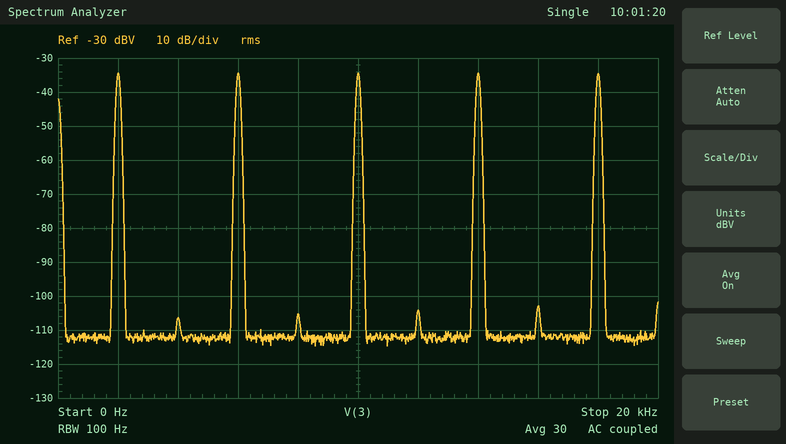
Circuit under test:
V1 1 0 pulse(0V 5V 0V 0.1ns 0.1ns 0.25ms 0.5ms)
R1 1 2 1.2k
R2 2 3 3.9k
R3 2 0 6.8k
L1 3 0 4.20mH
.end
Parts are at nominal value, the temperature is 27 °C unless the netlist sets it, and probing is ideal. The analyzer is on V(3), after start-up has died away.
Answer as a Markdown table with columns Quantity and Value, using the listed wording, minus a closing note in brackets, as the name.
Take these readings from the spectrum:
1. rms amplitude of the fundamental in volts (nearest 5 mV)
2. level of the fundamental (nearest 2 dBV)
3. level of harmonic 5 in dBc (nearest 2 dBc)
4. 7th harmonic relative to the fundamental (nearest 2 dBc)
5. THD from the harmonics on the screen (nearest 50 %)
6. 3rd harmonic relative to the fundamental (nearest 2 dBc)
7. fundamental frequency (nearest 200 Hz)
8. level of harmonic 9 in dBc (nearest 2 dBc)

| Quantity | Value |
|---|---|
| rms amplitude of the fundamental in volts | 20 mV |
| level of the fundamental | -34 dBV |
| level of harmonic 5 in dBc | 0 dBc |
| 7th harmonic relative to the fundamental | 0 dBc |
| THD from the harmonics on the screen | 200 % |
| 3rd harmonic relative to the fundamental | 0 dBc |
| fundamental frequency | 2.0 kHz |
| level of harmonic 9 in dBc | 0 dBc |
